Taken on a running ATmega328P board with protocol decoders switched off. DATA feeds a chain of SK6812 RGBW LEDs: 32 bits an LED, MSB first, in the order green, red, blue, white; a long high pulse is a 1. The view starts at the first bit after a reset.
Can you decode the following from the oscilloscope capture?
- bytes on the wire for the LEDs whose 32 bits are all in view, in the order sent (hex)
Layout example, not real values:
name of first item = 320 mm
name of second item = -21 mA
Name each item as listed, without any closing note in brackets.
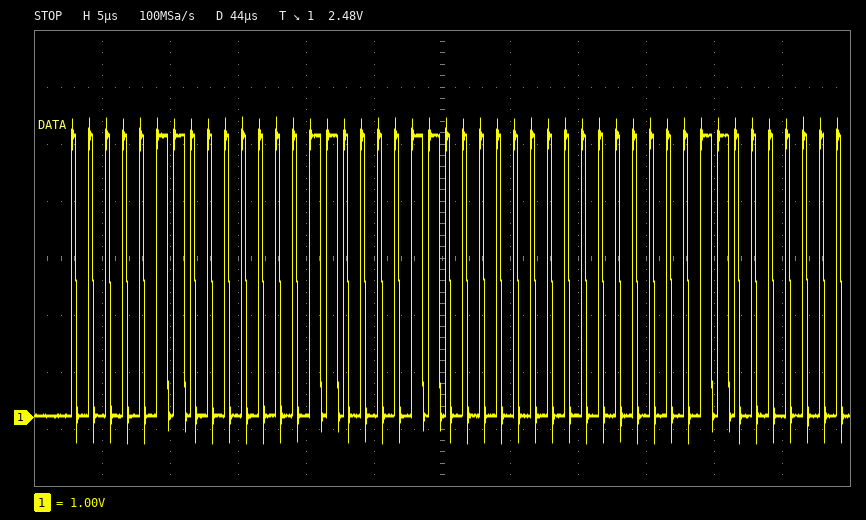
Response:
bytes on the wire for the LEDs whose 32 bits are all in view, in the order sent = 06 03 0C 00
